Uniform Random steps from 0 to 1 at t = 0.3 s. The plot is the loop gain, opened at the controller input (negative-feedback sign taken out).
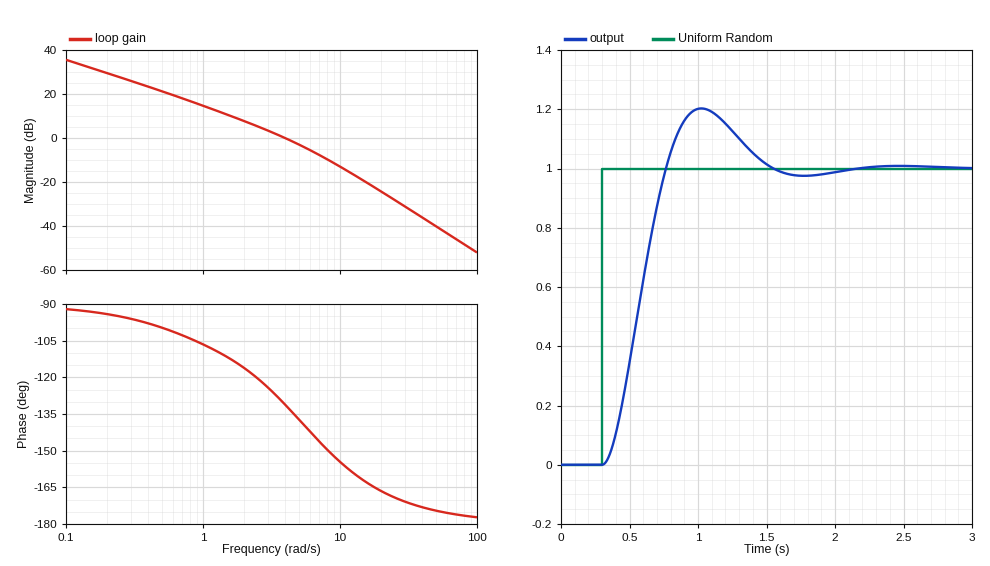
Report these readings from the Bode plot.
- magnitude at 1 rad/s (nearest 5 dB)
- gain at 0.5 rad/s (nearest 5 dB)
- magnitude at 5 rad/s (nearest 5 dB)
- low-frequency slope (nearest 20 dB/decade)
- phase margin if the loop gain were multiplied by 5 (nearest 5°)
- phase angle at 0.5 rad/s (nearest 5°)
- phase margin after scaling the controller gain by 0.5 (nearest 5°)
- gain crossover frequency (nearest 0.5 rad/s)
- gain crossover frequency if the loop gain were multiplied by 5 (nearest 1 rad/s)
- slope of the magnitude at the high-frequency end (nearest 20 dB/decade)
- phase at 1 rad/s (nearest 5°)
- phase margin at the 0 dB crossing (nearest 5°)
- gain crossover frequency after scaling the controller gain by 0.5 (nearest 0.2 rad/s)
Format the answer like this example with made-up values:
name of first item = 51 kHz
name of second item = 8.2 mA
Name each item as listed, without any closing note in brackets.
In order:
magnitude at 1 rad/s = 15 dB
gain at 0.5 rad/s = 20 dB
magnitude at 5 rad/s = -5 dB
low-frequency slope = -20 dB/decade
phase margin if the loop gain were multiplied by 5 = 25°
phase angle at 0.5 rad/s = -100°
phase margin after scaling the controller gain by 0.5 = 60°
gain crossover frequency = 4.0 rad/s
gain crossover frequency if the loop gain were multiplied by 5 = 11 rad/s
slope of the magnitude at the high-frequency end = -40 dB/decade
phase at 1 rad/s = -105°
phase margin at the 0 dB crossing = 50°
gain crossover frequency after scaling the controller gain by 0.5 = 2.4 rad/s
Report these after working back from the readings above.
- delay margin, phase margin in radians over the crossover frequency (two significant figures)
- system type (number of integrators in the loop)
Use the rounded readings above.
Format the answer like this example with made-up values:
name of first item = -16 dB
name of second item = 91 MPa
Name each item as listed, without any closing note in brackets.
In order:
delay margin, phase margin in radians over the crossover frequency = 0.22 s
system type = 1
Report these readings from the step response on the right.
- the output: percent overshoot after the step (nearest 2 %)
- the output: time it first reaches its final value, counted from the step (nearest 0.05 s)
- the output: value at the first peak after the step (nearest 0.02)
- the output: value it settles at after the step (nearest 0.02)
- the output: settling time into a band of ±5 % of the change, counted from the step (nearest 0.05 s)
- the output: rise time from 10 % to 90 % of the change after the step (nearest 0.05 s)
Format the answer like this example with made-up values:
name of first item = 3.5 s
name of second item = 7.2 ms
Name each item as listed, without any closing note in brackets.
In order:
the output: percent overshoot after the step = 20 %
the output: time it first reaches its final value, counted from the step = 0.45 s
the output: value at the first peak after the step = 1.20
the output: value it settles at after the step = 1.00
the output: settling time into a band of ±5 % of the change, counted from the step = 1.10 s
the output: rise time from 10 % to 90 % of the change after the step = 0.30 s
